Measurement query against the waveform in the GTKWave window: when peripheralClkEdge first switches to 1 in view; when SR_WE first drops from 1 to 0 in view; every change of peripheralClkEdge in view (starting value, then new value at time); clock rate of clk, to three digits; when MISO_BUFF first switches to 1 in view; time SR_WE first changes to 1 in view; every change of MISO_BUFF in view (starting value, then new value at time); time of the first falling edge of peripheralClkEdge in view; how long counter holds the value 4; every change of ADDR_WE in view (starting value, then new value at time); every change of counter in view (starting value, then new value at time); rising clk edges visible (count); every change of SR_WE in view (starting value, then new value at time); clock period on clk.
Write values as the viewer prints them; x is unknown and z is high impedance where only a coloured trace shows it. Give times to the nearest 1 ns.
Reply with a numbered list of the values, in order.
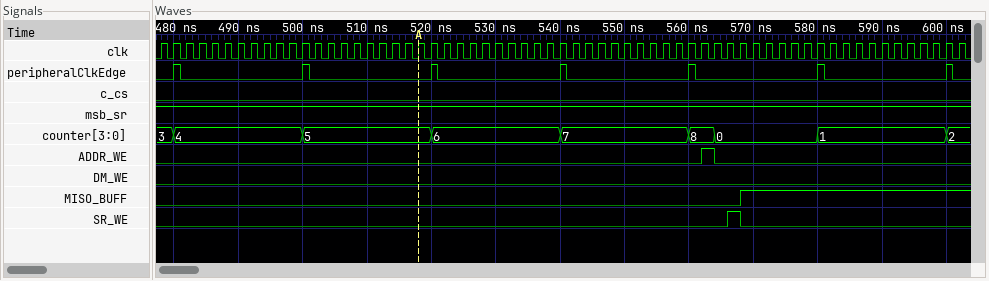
1. 480 ns
2. 568 ns
3. 0, 1 at 480 ns, 0 at 481 ns, 1 at 500 ns, 0 at 501 ns, 1 at 520 ns, 0 at 521 ns, 1 at 540 ns, 0 at 541 ns, 1 at 560 ns, 0 at 561 ns, 1 at 580 ns, 0 at 581 ns, 1 at 600 ns, 0 at 601 ns
4. 500 MHz
5. 568 ns
6. 566 ns
7. 0, 1 at 568 ns
8. 481 ns
9. 20 ns
10. 0, 1 at 562 ns, 0 at 564 ns
11. 3, 4 at 480 ns, 5 at 500 ns, 6 at 520 ns, 7 at 540 ns, 8 at 560 ns, 0 at 564 ns, 1 at 580 ns, 2 at 600 ns
12. 63
13. 0, 1 at 566 ns, 0 at 568 ns
14. 2 ns
